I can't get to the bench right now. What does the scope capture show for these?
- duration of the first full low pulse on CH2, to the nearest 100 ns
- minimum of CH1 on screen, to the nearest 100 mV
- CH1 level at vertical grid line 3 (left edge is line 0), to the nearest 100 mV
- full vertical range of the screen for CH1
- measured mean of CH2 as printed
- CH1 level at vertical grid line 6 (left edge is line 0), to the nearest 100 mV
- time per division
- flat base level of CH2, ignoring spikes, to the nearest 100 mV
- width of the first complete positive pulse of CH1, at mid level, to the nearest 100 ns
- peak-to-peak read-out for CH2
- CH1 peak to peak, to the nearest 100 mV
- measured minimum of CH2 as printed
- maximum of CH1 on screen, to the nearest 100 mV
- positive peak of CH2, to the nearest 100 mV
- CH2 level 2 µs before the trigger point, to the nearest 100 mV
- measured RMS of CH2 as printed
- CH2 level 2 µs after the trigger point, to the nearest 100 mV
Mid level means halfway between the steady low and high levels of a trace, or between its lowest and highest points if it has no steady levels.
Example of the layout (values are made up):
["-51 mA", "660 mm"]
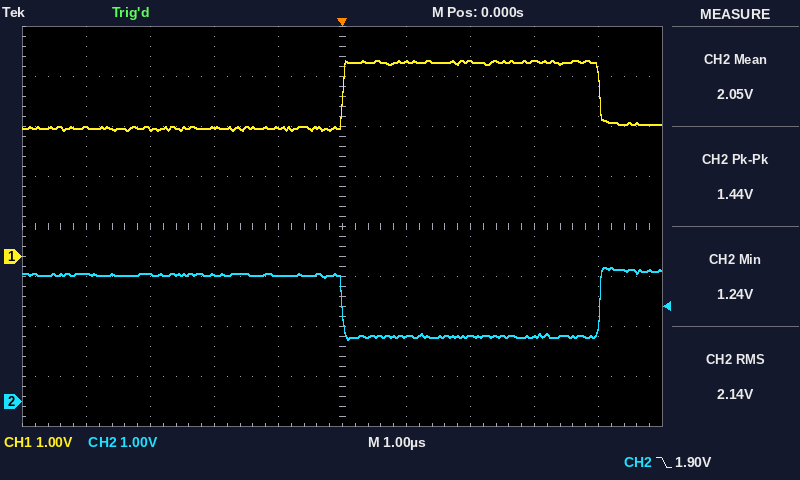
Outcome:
["4.0 µs", "2.5 V", "2.6 V", "8 V", "2.05 V", "3.9 V", "1 µs", "1.3 V", "4.0 µs", "1.44 V", "1.4 V", "1.24 V", "3.9 V", "2.7 V", "2.5 V", "2.14 V", "1.3 V"]
